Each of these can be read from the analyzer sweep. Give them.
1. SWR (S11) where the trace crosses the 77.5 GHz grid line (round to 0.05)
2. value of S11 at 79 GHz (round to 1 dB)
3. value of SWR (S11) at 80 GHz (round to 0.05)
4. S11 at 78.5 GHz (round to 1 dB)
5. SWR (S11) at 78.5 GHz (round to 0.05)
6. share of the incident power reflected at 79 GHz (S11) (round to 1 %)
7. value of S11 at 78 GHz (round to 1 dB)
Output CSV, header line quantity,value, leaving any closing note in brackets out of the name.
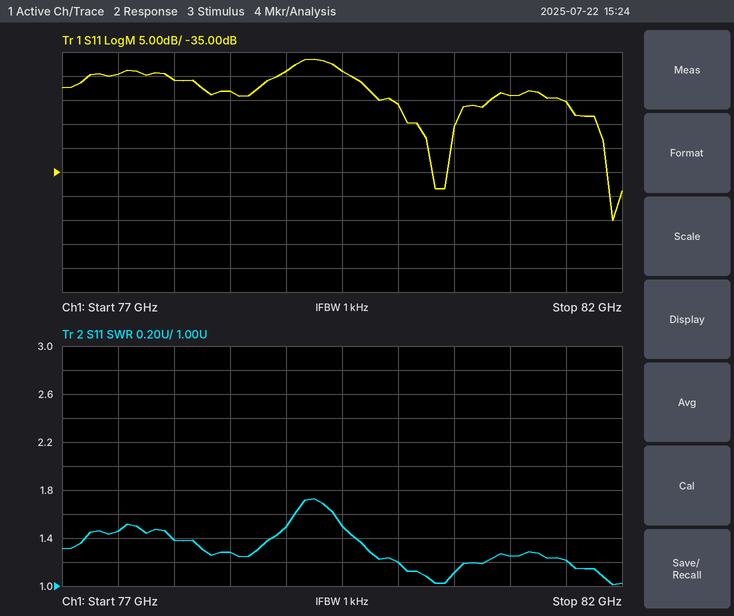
quantity,value
SWR (S11) where the trace crosses the 77.5 GHz grid line,1.45
value of S11 at 79 GHz,-14 dB
value of SWR (S11) at 80 GHz,1.20
S11 at 78.5 GHz,-18 dB
SWR (S11) at 78.5 GHz,1.30
share of the incident power reflected at 79 GHz (S11),4 %
value of S11 at 78 GHz,-16 dB
